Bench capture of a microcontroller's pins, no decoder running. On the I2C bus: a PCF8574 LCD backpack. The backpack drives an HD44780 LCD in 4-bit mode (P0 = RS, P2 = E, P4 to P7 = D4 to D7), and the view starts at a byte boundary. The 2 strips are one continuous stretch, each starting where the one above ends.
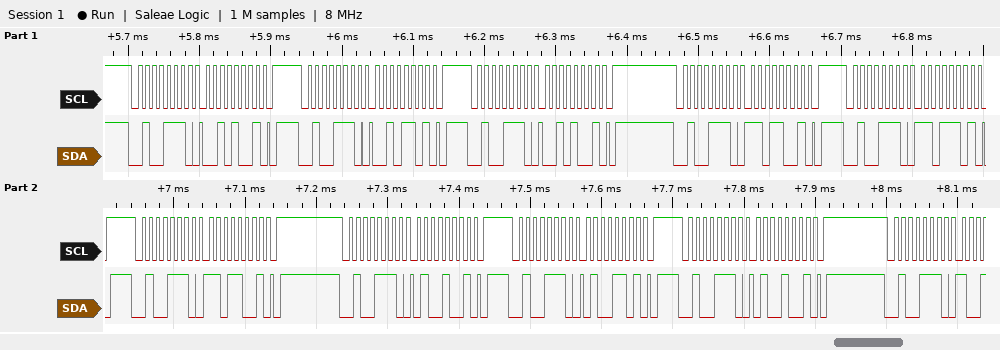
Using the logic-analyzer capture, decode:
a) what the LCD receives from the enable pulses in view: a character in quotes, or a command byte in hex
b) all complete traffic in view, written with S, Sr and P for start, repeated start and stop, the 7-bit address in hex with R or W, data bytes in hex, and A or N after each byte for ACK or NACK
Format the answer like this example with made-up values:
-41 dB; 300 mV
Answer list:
'-'; S 27W A 29 A P S 27W A 2D A P S 27W A 29 A P S 27W A D9 A P S 27W A DD A P S 27W A D9 A P S 27W A 49 A P S 27W A 4D A P S 27W A 49 A P S 27W A
